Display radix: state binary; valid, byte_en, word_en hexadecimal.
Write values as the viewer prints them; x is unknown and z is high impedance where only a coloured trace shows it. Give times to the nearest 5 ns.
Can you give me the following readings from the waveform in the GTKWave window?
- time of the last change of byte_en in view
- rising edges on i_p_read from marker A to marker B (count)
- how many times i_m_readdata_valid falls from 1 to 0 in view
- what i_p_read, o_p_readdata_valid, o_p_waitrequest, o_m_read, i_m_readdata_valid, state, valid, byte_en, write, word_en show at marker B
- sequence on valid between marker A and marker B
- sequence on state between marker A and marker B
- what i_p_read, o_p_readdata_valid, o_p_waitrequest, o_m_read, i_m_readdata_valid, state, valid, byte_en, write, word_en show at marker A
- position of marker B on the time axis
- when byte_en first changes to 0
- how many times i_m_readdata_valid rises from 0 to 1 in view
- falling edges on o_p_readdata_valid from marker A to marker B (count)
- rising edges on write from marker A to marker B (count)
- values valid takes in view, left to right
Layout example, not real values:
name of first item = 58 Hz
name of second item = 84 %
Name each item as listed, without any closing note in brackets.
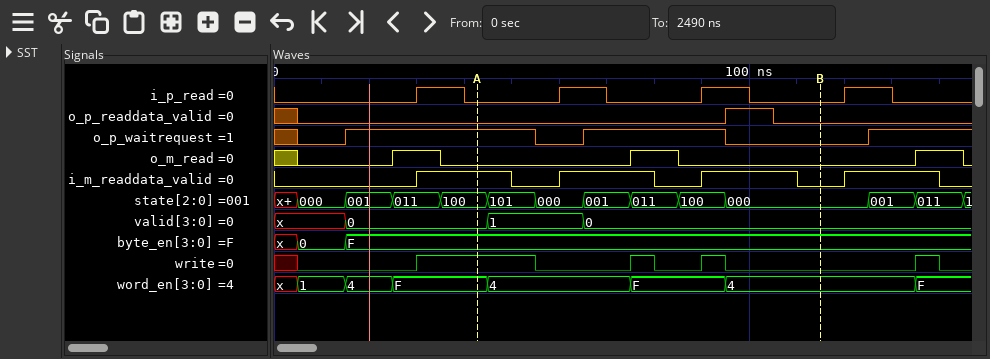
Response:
time of the last change of byte_en in view = 15 ns
rising edges on i_p_read from marker A to marker B = 2
how many times i_m_readdata_valid falls from 1 to 0 in view = 4
what i_p_read, o_p_readdata_valid, o_p_waitrequest, o_m_read, i_m_readdata_valid, state, valid, byte_en, write, word_en show at marker B = i_p_read=0, o_p_readdata_valid=0, o_p_waitrequest=0, o_m_read=0, i_m_readdata_valid=0, state=000, valid=0, byte_en=F, write=0, word_en=4
sequence on valid between marker A and marker B = 0, 1, 0
sequence on state between marker A and marker B = 100, 101, 000, 001, 011, 100, 000
what i_p_read, o_p_readdata_valid, o_p_waitrequest, o_m_read, i_m_readdata_valid, state, valid, byte_en, write, word_en show at marker A = i_p_read=0, o_p_readdata_valid=0, o_p_waitrequest=1, o_m_read=0, i_m_readdata_valid=1, state=100, valid=0, byte_en=F, write=1, word_en=F
position of marker B on the time axis = 115 ns
when byte_en first changes to 0 = 5 ns
how many times i_m_readdata_valid rises from 0 to 1 in view = 4
falling edges on o_p_readdata_valid from marker A to marker B = 1
rising edges on write from marker A to marker B = 2
values valid takes in view, left to right = x, 0, 1, 0
